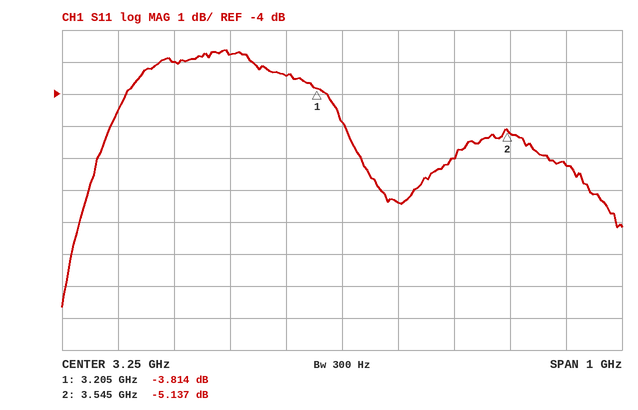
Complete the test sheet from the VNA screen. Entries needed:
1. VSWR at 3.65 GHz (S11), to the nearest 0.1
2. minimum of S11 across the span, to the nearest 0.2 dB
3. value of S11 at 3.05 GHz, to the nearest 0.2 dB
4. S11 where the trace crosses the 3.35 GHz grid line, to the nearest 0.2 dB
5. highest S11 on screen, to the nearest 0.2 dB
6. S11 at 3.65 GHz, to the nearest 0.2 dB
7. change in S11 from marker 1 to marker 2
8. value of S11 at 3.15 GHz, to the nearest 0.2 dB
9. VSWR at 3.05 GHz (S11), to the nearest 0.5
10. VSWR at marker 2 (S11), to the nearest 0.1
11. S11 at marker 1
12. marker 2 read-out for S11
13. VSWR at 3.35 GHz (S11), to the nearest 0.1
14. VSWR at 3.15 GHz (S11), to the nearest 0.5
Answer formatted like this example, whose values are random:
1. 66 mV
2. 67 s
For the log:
1. 2.9
2. -10.6 dB
3. -2.8 dB
4. -7.4 dB
5. -2.6 dB
6. -6.2 dB
7. -1.323 dB
8. -3.4 dB
9. 6.5
10. 3.5
11. -3.814 dB
12. -5.137 dB
13. 2.5
14. 5.0
